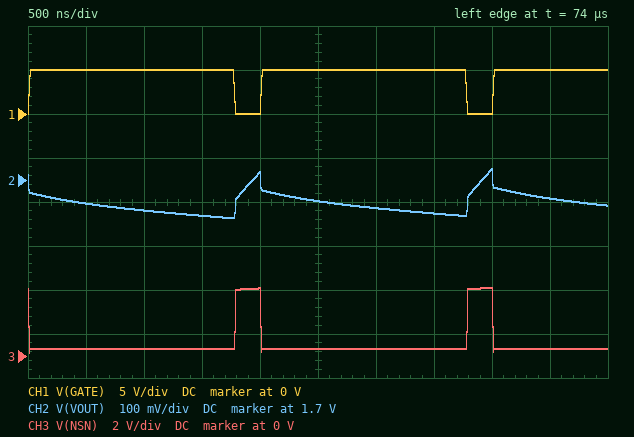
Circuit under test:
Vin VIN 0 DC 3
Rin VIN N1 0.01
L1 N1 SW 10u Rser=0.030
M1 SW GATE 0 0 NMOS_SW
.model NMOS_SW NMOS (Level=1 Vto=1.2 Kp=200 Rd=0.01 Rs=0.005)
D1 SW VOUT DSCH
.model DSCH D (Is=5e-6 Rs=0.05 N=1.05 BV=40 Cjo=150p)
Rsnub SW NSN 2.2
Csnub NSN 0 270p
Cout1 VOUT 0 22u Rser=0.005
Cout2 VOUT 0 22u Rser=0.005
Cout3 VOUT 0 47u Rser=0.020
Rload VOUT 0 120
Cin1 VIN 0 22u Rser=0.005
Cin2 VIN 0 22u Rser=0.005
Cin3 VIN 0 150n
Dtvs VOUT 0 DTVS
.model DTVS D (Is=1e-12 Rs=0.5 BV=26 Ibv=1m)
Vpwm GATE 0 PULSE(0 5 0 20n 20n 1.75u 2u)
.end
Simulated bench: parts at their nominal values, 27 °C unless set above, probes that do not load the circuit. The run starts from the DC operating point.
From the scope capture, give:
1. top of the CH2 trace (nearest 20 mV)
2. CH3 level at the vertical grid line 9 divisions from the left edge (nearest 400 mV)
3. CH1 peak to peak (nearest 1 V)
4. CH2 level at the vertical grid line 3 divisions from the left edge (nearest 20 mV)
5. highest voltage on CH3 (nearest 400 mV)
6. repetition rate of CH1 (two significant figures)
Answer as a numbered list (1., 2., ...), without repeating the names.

1. 1.72 V
2. 400 mV
3. 5 V
4. 1.62 V
5. 3.2 V
6. 500 kHz
